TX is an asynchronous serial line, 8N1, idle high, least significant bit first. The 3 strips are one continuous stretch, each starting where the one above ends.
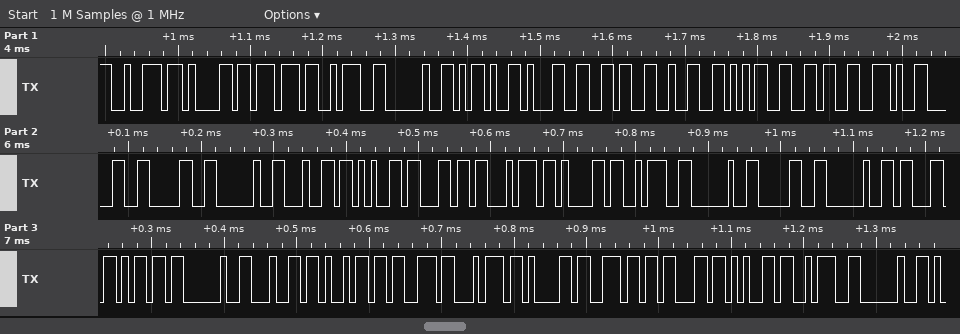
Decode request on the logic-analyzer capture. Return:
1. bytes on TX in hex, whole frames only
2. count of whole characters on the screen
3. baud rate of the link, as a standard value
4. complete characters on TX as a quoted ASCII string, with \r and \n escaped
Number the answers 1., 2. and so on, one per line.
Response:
1. 72 61 77 3A 20 2D 31 36 32 35 36 2E 30 30 20 64 65 6C 74 61 3A 20 30 20 63 6D 20 64 69 73 74 61 6E 63 65 3A 20
2. 37
3. 115200 baud
4. "raw: -16256.00 delta: 0 cm distance: "
